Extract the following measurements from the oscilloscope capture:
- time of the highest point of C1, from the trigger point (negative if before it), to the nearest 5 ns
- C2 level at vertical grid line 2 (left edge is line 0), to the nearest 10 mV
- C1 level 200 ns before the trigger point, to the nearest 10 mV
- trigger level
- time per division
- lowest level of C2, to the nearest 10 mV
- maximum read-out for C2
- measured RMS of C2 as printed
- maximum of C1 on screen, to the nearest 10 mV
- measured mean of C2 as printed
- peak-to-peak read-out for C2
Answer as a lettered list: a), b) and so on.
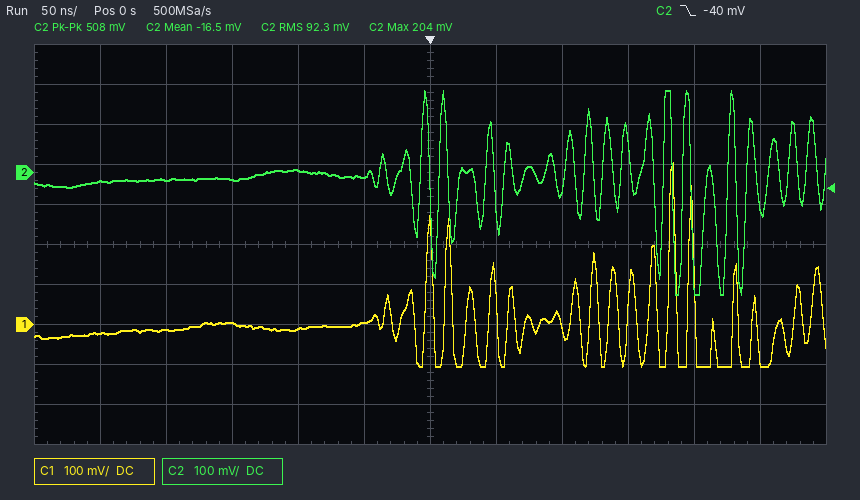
a) +185 ns
b) -20 mV
c) -10 mV
d) -40 mV
e) 50 ns
f) -300 mV
g) 204 mV
h) 92.3 mV
i) 400 mV
j) -16.5 mV
k) 508 mV
